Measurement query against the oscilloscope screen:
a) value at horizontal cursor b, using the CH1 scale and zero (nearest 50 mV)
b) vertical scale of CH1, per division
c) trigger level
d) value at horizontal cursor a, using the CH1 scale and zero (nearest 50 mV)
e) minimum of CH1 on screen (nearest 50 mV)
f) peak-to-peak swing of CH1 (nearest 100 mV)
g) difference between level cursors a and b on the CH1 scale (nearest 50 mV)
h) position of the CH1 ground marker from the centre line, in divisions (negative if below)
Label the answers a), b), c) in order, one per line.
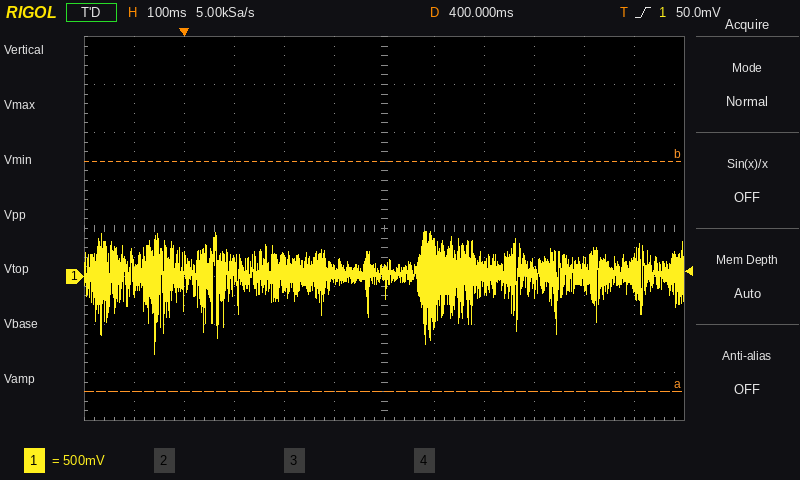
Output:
a) 1.20 V
b) 500 mV
c) 50.0 mV
d) -1.20 V
e) -800 mV
f) 1.30 V
g) 2.40 V
h) -1.0 div
